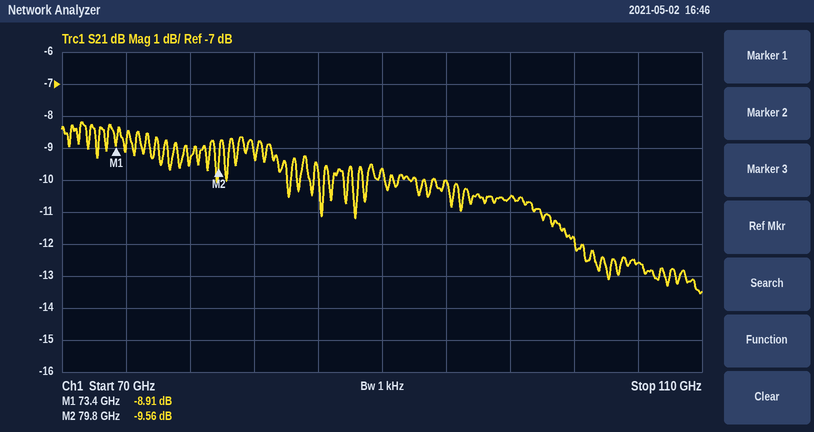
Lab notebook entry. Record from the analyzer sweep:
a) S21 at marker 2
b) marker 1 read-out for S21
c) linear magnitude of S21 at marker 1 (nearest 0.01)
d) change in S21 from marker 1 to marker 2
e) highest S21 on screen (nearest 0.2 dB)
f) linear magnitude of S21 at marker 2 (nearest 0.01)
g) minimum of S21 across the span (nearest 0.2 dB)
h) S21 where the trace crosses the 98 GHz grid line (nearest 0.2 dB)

-9.56 dB
-8.91 dB
0.36
-0.65 dB
-8.2 dB
0.33
-13.6 dB
-10.6 dB
